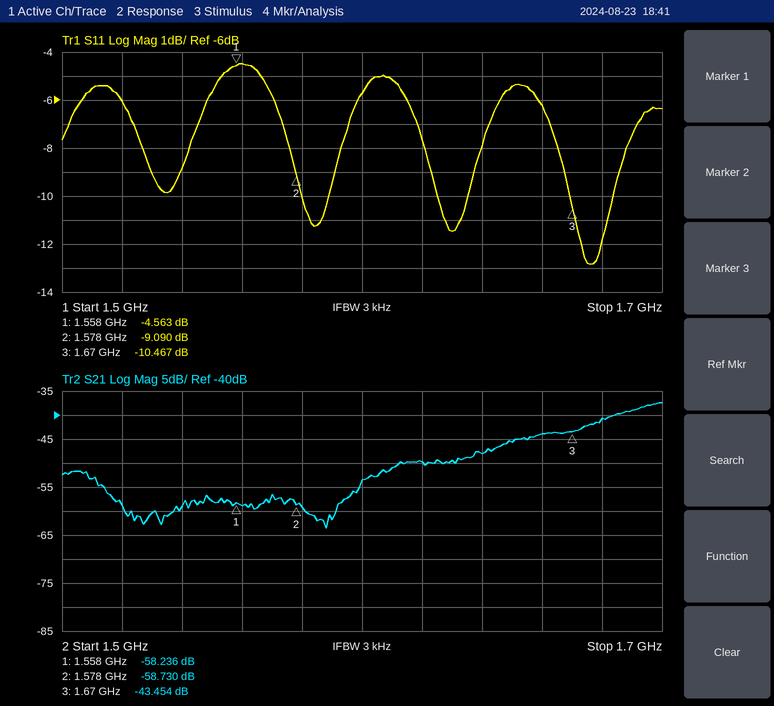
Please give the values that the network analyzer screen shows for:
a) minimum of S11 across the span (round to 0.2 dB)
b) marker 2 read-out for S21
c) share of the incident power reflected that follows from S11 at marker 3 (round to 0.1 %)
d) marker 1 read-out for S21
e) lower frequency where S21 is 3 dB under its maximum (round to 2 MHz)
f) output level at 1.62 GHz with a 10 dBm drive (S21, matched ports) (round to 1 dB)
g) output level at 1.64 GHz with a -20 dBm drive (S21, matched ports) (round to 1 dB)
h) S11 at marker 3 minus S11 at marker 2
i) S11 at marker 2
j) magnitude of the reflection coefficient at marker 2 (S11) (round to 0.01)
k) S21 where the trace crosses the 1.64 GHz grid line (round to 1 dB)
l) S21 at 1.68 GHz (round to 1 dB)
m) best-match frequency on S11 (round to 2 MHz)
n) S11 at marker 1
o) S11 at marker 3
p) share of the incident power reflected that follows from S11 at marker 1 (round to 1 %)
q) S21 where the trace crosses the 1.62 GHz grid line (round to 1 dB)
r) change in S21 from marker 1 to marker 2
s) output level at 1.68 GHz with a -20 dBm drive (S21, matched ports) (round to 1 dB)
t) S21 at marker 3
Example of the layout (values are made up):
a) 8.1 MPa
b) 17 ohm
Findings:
a) -12.8 dB
b) -58.730 dB
c) 9.0 %
d) -58.236 dB
e) 1.682 GHz
f) -40 dBm
g) -68 dBm
h) -1.377 dB
i) -9.090 dB
j) 0.35
k) -48 dB
l) -41 dB
m) 1.676 GHz
n) -4.563 dB
o) -10.467 dB
p) 35 %
q) -50 dB
r) -0.494 dB
s) -61 dBm
t) -43.454 dB
